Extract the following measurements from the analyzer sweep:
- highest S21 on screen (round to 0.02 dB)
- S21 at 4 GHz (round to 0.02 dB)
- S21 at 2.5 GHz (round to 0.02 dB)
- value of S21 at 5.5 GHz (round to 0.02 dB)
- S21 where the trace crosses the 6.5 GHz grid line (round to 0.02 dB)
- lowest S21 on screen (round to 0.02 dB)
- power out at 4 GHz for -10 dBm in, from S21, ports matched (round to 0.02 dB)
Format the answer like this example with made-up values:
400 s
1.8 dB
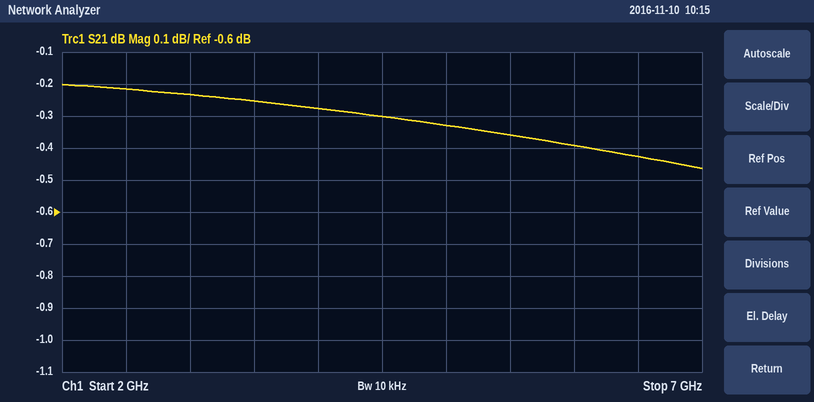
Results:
-0.20 dB
-0.28 dB
-0.22 dB
-0.36 dB
-0.42 dB
-0.46 dB
-10.28 dBm
